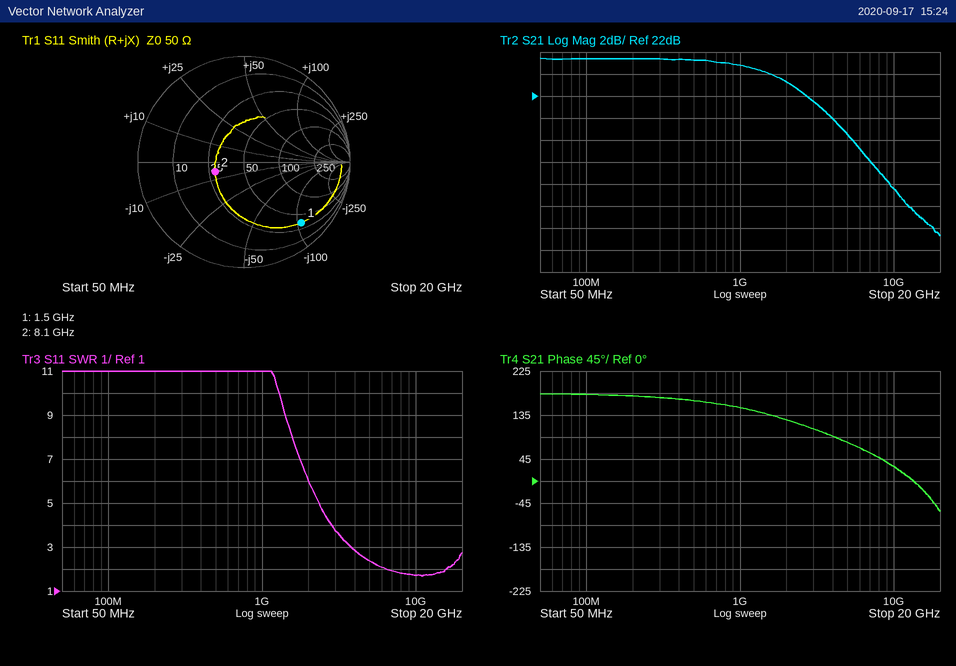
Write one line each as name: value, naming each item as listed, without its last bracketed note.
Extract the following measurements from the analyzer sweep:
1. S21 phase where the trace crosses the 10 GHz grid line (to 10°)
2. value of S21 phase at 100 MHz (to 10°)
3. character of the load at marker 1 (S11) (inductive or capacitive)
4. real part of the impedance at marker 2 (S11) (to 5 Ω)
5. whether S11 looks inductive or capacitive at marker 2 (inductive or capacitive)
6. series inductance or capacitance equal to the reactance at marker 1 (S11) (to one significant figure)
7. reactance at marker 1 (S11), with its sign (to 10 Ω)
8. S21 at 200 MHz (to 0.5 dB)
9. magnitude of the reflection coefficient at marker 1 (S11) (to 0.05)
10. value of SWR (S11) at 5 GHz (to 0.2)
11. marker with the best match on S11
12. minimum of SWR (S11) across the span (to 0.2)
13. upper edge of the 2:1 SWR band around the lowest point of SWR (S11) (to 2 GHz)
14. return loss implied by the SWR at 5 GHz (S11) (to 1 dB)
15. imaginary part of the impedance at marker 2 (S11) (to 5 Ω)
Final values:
S21 phase where the trace crosses the 10 GHz grid line: 30°
value of S21 phase at 100 MHz: 180°
character of the load at marker 1 (S11): capacitive
real part of the impedance at marker 2 (S11): 30 Ω
whether S11 looks inductive or capacitive at marker 2: capacitive
series inductance or capacitance equal to the reactance at marker 1 (S11): 1.0 pF
reactance at marker 1 (S11), with its sign: -110 Ω
S21 at 200 MHz: 25.5 dB
magnitude of the reflection coefficient at marker 1 (S11): 0.80
value of SWR (S11) at 5 GHz: 2.4
marker with the best match on S11: marker 2
minimum of SWR (S11) across the span: 1.6
upper edge of the 2:1 SWR band around the lowest point of SWR (S11): 16 GHz
return loss implied by the SWR at 5 GHz (S11): 8 dB
imaginary part of the impedance at marker 2 (S11): -5 Ω
